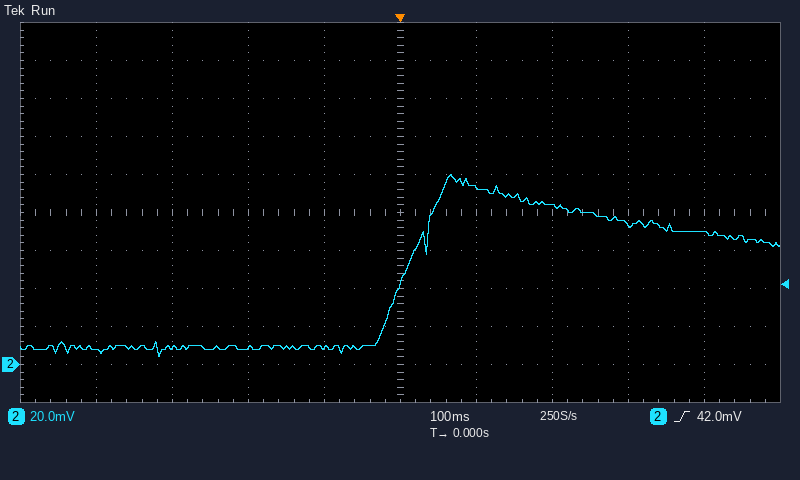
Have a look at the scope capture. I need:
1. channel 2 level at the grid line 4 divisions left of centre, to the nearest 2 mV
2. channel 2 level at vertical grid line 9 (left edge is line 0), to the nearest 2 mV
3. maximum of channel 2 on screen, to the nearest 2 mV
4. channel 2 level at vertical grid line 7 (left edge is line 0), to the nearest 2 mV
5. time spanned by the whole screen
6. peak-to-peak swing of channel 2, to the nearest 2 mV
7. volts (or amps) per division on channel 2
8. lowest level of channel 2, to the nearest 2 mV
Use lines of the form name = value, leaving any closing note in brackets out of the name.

channel 2 level at the grid line 4 divisions left of centre, to the nearest 2 mV = 8 mV
channel 2 level at vertical grid line 9 (left edge is line 0), to the nearest 2 mV = 70 mV
maximum of channel 2 on screen, to the nearest 2 mV = 100 mV
channel 2 level at vertical grid line 7 (left edge is line 0), to the nearest 2 mV = 84 mV
time spanned by the whole screen = 1 s
peak-to-peak swing of channel 2, to the nearest 2 mV = 96 mV
volts (or amps) per division on channel 2 = 20 mV
lowest level of channel 2, to the nearest 2 mV = 4 mV
